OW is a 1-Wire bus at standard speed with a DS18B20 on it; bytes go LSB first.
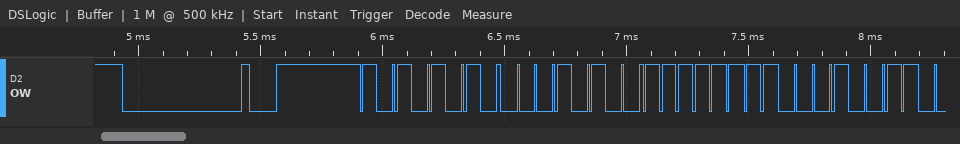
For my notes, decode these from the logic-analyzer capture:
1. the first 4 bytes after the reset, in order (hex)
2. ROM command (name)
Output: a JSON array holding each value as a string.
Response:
["55 28 FF C8", "Match ROM"]
